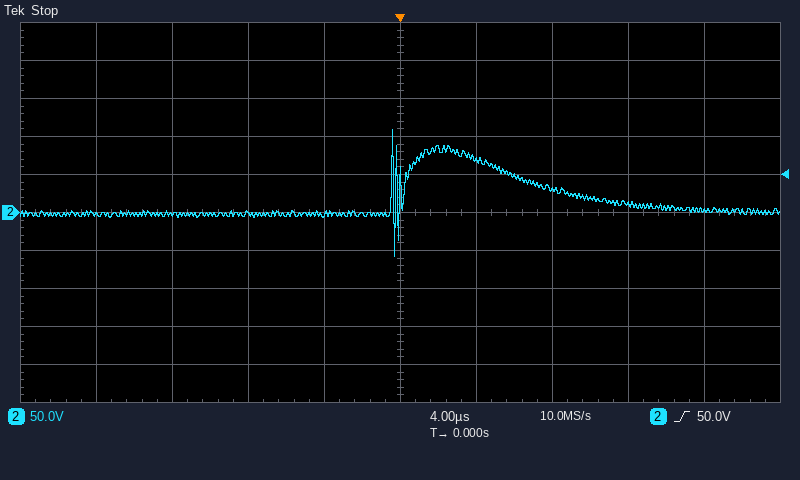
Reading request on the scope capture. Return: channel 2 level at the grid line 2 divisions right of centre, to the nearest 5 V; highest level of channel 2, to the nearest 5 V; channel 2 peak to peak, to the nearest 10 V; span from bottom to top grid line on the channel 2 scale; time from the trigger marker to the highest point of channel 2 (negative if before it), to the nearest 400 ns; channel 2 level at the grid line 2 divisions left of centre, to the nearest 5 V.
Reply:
30 V
110 V
170 V
500 V
-400 ns
0 V
